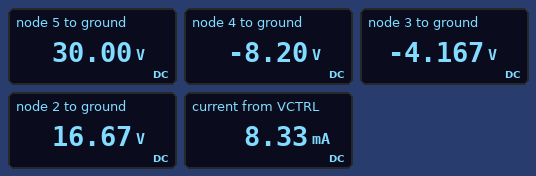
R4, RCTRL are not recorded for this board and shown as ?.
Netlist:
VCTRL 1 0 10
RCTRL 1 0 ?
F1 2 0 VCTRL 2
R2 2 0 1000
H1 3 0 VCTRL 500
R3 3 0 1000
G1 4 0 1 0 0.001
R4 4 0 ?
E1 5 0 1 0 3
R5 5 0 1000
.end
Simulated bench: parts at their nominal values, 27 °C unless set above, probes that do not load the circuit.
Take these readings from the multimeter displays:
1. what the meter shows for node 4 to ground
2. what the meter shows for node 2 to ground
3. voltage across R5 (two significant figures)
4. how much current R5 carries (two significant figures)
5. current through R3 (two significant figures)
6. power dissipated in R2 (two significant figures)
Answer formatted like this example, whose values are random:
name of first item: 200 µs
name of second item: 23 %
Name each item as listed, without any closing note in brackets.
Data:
what the meter shows for node 4 to ground: -8.20 V
what the meter shows for node 2 to ground: 16.67 V
voltage across R5: 30 V
how much current R5 carries: 30 mA
current through R3: 4.2 mA
power dissipated in R2: 280 mW
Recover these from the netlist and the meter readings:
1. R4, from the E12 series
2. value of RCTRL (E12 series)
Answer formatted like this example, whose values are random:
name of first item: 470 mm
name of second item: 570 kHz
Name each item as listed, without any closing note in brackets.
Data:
R4, from the E12 series: 820 Ω
value of RCTRL: 1.2 kΩ
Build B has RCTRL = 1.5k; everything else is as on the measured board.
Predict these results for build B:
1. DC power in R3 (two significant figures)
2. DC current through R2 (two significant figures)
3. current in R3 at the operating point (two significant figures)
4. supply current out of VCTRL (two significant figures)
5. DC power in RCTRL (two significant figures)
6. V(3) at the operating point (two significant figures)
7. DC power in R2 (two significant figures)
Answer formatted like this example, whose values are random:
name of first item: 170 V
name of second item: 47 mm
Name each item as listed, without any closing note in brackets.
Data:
DC power in R3: 11 mW
DC current through R2: 13 mA
current in R3 at the operating point: 3.3 mA
supply current out of VCTRL: 6.7 mA
DC power in RCTRL: 67 mW
V(3) at the operating point: -3.3 V
DC power in R2: 180 mW
